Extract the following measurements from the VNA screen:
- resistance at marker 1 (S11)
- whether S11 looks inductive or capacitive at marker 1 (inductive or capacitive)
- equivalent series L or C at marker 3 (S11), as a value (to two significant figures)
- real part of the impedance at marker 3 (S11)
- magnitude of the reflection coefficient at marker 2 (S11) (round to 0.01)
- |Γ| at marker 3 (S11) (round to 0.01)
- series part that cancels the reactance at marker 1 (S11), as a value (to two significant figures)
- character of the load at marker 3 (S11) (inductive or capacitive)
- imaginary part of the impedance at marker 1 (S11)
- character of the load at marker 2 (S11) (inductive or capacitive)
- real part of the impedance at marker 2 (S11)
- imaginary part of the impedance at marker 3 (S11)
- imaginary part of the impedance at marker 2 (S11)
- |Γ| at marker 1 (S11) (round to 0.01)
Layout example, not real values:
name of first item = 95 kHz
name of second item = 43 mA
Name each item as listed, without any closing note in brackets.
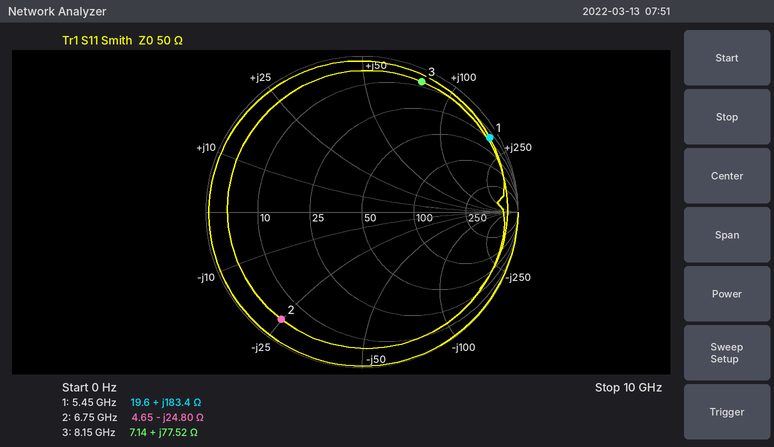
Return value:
resistance at marker 1 = 19.6 Ω
whether S11 looks inductive or capacitive at marker 1 = inductive
equivalent series L or C at marker 3 (S11), as a value = 1.5 nH
real part of the impedance at marker 3 = 7.14 Ω
magnitude of the reflection coefficient at marker 2 (S11) = 0.86
|Γ| at marker 3 (S11) = 0.92
series part that cancels the reactance at marker 1 (S11), as a value = 160 fF
character of the load at marker 3 (S11) = inductive
imaginary part of the impedance at marker 1 = +183.4 Ω
character of the load at marker 2 (S11) = capacitive
real part of the impedance at marker 2 = 4.65 Ω
imaginary part of the impedance at marker 3 = +77.52 Ω
imaginary part of the impedance at marker 2 = -24.80 Ω
|Γ| at marker 1 (S11) = 0.95
